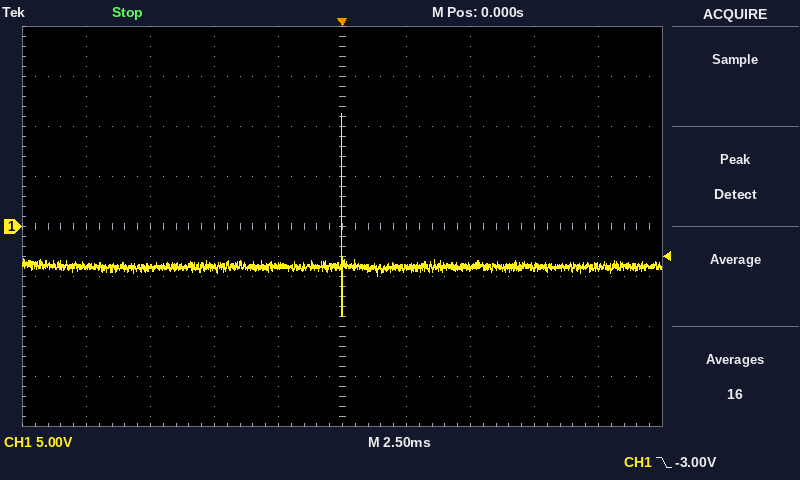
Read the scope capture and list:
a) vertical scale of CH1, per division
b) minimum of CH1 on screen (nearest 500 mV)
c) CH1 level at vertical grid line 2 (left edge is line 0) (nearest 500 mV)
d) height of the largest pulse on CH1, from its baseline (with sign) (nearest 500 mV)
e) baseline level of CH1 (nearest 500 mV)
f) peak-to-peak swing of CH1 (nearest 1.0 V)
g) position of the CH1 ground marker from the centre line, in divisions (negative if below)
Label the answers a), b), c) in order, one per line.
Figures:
a) 5 V
b) -9.0 V
c) -4.0 V
d) +15.5 V
e) -4.0 V
f) 20.0 V
g) 0.0 div
